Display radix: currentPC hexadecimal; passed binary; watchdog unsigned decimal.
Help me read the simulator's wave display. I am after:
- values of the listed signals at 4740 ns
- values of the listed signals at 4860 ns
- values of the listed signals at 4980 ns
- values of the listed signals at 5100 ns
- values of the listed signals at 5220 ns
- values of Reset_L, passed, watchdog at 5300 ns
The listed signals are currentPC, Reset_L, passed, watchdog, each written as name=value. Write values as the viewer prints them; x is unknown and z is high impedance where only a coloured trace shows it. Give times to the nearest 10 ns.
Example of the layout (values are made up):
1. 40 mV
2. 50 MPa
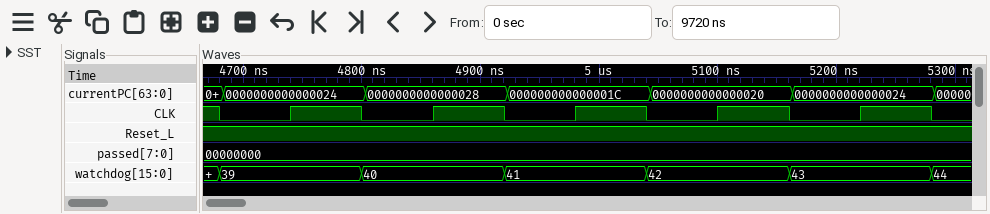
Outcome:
1. currentPC=0000000000000024, Reset_L=1, passed=00000000, watchdog=39
2. currentPC=0000000000000028, Reset_L=1, passed=00000000, watchdog=40
3. currentPC=000000000000001C, Reset_L=1, passed=00000000, watchdog=41
4. currentPC=0000000000000020, Reset_L=1, passed=00000000, watchdog=42
5. currentPC=0000000000000024, Reset_L=1, passed=00000000, watchdog=43
6. Reset_L=1, passed=00000000, watchdog=44
